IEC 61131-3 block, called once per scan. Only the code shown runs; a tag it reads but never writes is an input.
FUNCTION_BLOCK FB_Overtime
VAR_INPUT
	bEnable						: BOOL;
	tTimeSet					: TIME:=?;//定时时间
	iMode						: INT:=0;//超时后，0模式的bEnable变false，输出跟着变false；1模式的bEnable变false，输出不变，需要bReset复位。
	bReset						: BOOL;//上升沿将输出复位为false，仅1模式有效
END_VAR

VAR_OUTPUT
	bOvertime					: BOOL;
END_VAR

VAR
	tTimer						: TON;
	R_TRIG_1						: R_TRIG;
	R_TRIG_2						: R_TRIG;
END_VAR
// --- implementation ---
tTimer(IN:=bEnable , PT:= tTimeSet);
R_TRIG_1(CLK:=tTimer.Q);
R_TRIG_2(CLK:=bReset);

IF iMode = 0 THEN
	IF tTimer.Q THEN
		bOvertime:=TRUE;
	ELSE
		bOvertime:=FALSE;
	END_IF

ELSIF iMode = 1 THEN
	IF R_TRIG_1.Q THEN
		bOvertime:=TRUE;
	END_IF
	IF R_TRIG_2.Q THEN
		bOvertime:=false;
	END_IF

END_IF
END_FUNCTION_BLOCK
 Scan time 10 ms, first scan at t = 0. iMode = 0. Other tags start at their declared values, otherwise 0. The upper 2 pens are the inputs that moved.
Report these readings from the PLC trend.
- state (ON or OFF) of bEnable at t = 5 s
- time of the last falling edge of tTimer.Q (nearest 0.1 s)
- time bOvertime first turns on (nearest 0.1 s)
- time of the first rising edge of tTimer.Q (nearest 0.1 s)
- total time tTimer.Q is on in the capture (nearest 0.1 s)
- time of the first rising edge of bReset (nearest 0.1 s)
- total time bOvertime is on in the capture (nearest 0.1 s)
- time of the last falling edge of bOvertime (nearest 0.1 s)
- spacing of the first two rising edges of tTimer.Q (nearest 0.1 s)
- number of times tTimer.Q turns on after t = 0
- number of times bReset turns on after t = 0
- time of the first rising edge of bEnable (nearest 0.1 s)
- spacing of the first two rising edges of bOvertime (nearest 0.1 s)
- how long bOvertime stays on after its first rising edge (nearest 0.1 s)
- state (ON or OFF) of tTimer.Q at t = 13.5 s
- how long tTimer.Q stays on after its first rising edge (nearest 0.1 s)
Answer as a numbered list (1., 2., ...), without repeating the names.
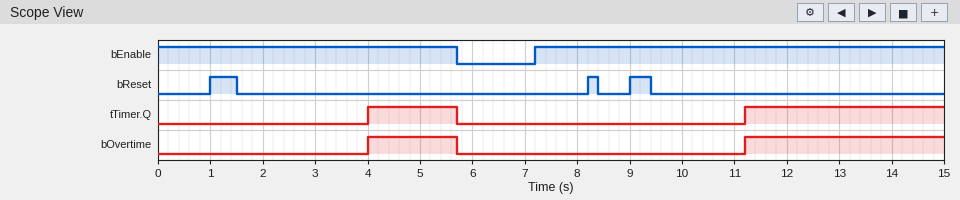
1. ON
2. 5.7 s
3. 4.0 s
4. 4.0 s
5. 5.5 s
6. 1.0 s
7. 5.5 s
8. 5.7 s
9. 7.2 s
10. 2
11. 3
12. 7.2 s
13. 7.2 s
14. 1.7 s
15. ON
16. 1.7 s
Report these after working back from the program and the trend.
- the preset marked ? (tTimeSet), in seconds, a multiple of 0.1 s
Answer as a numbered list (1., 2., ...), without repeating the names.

1. 4.0 s
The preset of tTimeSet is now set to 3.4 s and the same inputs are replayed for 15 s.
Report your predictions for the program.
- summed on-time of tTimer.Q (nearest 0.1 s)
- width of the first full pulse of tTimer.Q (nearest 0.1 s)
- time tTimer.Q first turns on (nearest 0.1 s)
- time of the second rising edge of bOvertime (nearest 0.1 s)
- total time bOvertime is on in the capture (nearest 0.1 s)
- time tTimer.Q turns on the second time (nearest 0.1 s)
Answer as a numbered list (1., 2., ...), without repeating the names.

1. 6.7 s
2. 2.3 s
3. 3.4 s
4. 10.6 s
5. 6.7 s
6. 10.6 s
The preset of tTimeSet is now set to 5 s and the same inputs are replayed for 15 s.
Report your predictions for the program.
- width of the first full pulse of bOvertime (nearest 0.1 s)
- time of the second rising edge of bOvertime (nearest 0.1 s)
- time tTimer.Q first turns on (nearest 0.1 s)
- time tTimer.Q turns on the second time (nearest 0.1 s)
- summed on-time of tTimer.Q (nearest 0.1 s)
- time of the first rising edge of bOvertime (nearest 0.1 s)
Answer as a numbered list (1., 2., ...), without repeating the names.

1. 0.7 s
2. 12.2 s
3. 5.0 s
4. 12.2 s
5. 3.5 s
6. 5.0 s
